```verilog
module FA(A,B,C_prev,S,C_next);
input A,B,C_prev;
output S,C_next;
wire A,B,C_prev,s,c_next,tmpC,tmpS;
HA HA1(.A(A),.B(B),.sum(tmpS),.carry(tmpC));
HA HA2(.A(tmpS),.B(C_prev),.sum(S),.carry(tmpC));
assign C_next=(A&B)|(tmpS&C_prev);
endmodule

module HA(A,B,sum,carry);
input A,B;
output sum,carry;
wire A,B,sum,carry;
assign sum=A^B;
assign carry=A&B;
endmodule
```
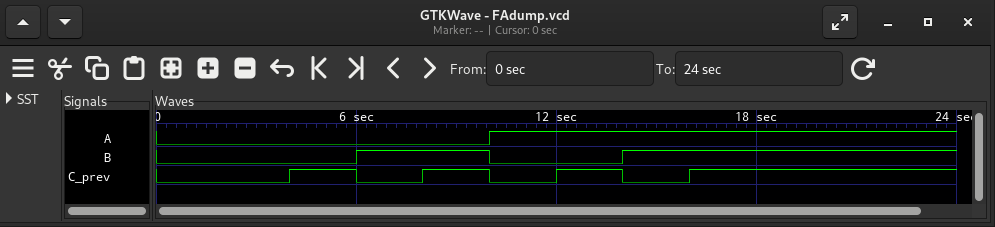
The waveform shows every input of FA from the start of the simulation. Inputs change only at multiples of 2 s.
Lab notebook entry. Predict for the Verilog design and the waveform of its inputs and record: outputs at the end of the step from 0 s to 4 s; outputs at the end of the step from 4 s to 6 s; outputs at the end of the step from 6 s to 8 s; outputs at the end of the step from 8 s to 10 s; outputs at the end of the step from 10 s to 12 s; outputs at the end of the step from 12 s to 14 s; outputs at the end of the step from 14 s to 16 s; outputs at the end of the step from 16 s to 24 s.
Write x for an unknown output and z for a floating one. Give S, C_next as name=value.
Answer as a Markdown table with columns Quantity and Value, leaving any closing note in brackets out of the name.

| Quantity | Value |
|---|---|
| outputs at the end of the step from 0 s to 4 s | S=0, C_next=0 |
| outputs at the end of the step from 4 s to 6 s | S=1, C_next=0 |
| outputs at the end of the step from 6 s to 8 s | S=1, C_next=0 |
| outputs at the end of the step from 8 s to 10 s | S=0, C_next=1 |
| outputs at the end of the step from 10 s to 12 s | S=1, C_next=0 |
| outputs at the end of the step from 12 s to 14 s | S=0, C_next=1 |
| outputs at the end of the step from 14 s to 16 s | S=0, C_next=1 |
| outputs at the end of the step from 16 s to 24 s | S=1, C_next=1 |
